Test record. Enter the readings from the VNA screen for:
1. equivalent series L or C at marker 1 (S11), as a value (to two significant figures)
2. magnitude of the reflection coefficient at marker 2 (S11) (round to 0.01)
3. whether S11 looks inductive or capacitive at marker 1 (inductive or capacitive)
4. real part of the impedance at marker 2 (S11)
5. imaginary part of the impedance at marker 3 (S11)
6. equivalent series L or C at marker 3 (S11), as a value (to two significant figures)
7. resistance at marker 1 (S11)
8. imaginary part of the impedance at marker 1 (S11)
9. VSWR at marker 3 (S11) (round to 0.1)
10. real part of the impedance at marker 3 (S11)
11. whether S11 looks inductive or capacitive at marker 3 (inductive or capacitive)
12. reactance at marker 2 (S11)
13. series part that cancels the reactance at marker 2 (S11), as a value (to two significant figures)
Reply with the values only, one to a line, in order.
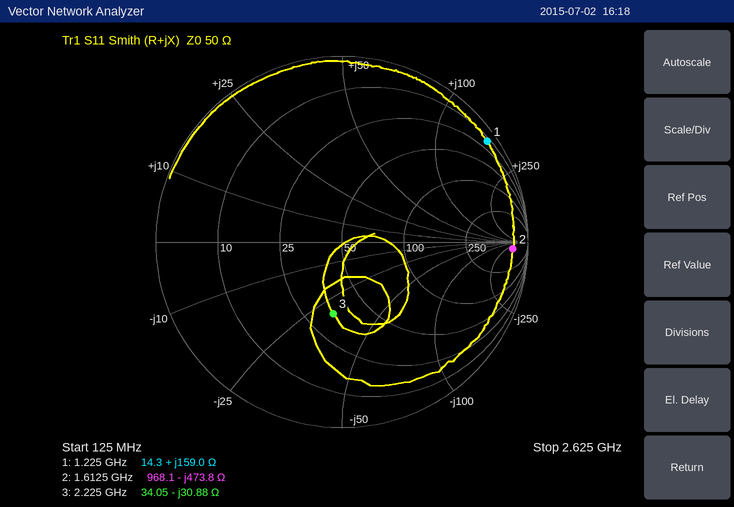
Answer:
21 nH
0.92
inductive
968.1 Ω
-30.88 Ω
2.3 pF
14.3 Ω
+159.0 Ω
2.3
34.05 Ω
capacitive
-473.8 Ω
47 nH
